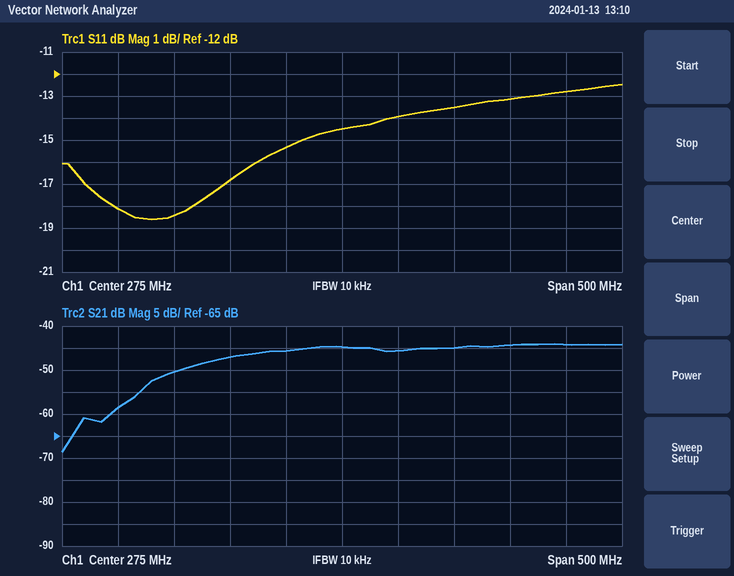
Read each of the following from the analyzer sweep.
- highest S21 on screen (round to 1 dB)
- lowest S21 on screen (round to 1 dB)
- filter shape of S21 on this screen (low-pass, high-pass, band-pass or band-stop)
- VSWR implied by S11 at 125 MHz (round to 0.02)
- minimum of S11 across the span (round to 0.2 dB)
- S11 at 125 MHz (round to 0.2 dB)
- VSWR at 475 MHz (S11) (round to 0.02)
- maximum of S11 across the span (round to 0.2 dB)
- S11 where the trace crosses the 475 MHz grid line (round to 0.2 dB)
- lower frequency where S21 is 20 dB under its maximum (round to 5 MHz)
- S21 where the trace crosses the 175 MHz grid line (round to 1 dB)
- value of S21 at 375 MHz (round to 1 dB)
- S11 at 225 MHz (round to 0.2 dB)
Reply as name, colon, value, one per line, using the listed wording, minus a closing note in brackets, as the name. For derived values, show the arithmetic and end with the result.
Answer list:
highest S21 on screen: -44 dB
lowest S21 on screen: -69 dB
filter shape of S21 on this screen: high-pass
VSWR implied by S11 at 125 MHz: |Γ| = 10^(-18.4/20) = 0.1202; VSWR = (1 + 0.1202)/(1 − 0.1202) ≈ 1.27, so 1.28 to the nearest 0.02
minimum of S11 across the span: -18.6 dB
S11 at 125 MHz: -18.4 dB
VSWR at 475 MHz (S11): |Γ| = 10^(-12.8/20) = 0.2291; VSWR = (1 + 0.2291)/(1 − 0.2291) ≈ 1.59, so 1.60 to the nearest 0.02
maximum of S11 across the span: -12.4 dB
S11 where the trace crosses the 475 MHz grid line: -12.8 dB
lower frequency where S21 is 20 dB under its maximum: 35 MHz
S21 where the trace crosses the 175 MHz grid line: -47 dB
value of S21 at 375 MHz: -45 dB
S11 at 225 MHz: -15.4 dB
